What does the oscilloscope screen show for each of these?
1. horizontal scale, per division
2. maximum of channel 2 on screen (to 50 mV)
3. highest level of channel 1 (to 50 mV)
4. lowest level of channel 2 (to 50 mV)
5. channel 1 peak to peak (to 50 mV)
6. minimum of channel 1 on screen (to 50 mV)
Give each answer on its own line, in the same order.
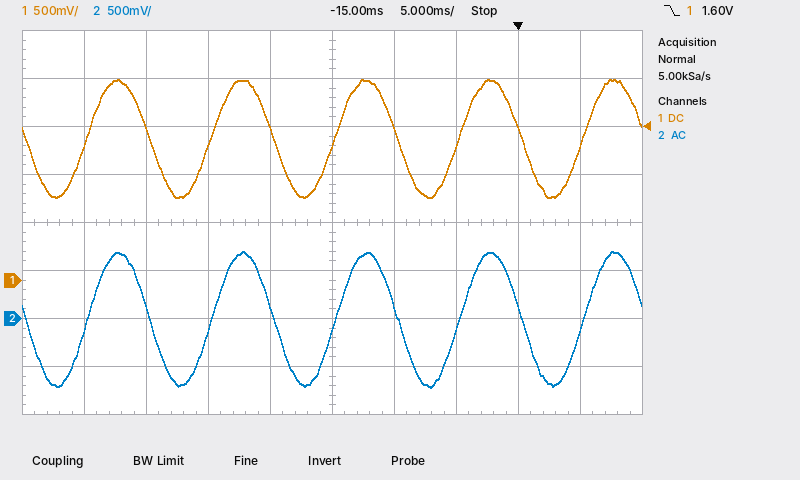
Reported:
5 ms
700 mV
2.10 V
-700 mV
1.25 V
850 mV
